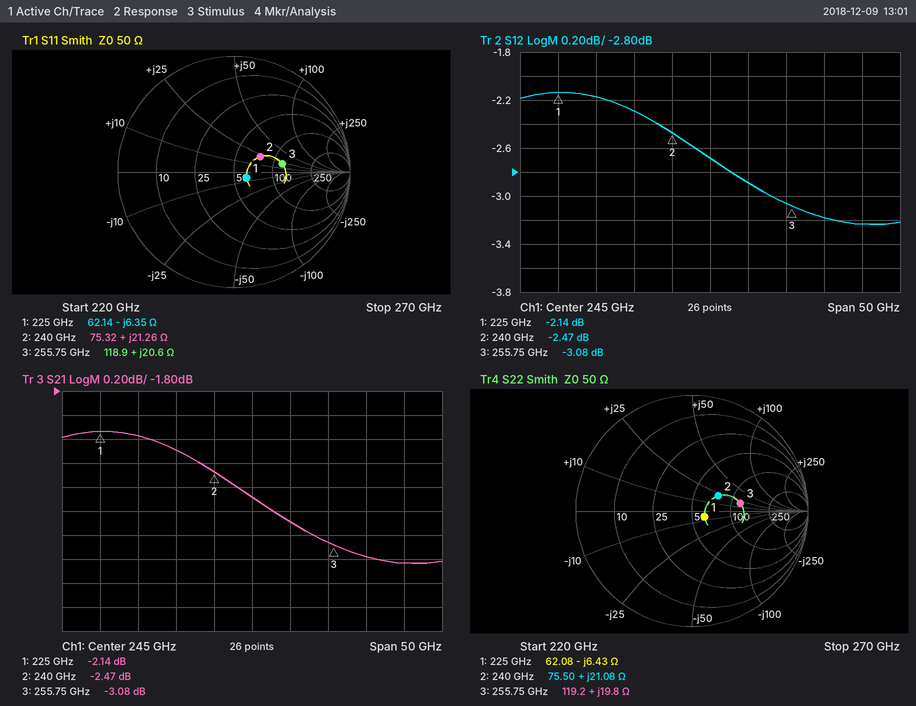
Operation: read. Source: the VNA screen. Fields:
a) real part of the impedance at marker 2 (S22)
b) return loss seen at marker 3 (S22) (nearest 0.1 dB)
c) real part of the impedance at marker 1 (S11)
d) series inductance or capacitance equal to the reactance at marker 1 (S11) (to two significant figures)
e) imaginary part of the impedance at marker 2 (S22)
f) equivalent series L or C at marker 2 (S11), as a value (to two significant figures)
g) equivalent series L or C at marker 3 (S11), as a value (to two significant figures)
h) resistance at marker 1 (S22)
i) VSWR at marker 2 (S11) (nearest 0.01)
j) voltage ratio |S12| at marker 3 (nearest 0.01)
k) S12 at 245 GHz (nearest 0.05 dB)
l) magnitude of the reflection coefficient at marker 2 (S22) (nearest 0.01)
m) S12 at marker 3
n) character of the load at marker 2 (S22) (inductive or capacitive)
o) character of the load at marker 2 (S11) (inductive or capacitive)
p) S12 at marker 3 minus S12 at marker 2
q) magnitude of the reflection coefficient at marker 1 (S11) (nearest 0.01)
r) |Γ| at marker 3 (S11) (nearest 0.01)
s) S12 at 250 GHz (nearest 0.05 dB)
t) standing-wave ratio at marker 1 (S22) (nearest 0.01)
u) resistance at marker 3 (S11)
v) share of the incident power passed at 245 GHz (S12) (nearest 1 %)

75.50 Ω
7.5 dB
62.14 Ω
110 fF
+21.08 Ω
14 pH
13 pH
62.08 Ω
1.70
0.70
-2.70 dB
0.26
-3.08 dB
inductive
inductive
-0.61 dB
0.12
0.42
-2.90 dB
1.28
118.9 Ω
54 %
